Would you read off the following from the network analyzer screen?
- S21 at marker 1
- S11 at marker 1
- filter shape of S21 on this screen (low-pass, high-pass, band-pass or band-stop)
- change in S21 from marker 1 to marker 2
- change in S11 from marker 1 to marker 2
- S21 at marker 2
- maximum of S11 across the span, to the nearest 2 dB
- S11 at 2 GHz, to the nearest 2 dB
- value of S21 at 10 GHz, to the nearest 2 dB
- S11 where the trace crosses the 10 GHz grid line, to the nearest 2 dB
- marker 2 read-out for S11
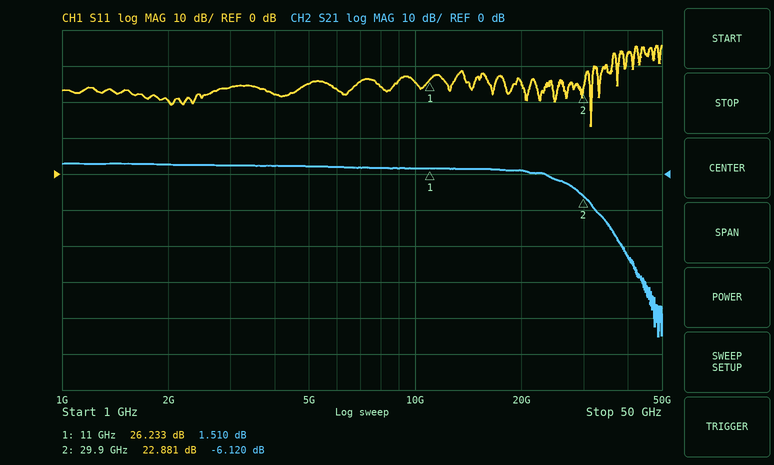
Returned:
1.510 dB
26.233 dB
low-pass
-7.630 dB
-3.352 dB
-6.120 dB
36 dB
20 dB
2 dB
26 dB
22.881 dB
